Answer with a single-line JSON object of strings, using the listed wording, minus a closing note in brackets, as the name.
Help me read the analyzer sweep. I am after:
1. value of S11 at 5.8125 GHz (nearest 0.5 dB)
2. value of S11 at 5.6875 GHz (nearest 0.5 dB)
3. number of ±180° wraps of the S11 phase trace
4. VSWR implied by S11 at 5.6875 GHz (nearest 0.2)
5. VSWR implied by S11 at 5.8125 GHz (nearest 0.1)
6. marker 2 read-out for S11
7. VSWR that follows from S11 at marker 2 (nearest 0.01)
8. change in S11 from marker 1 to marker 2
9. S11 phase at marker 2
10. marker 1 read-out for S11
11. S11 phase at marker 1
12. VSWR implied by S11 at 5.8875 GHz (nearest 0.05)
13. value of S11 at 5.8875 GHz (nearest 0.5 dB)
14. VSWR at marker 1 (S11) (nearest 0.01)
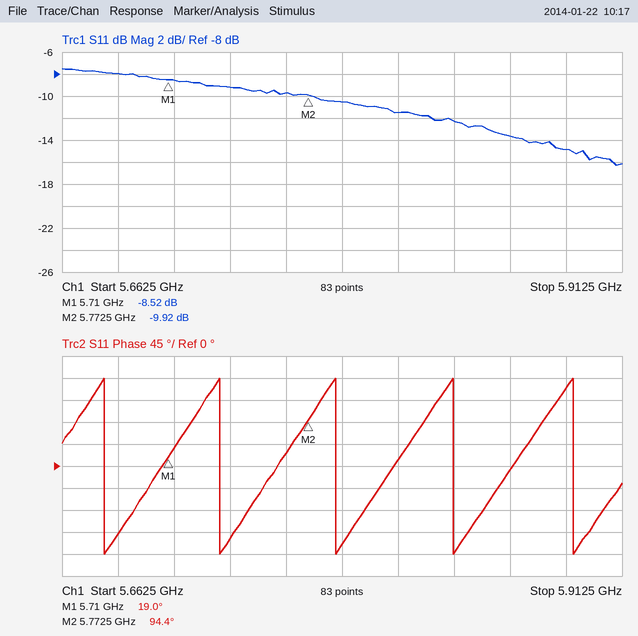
{"value of S11 at 5.8125 GHz": "-11.5 dB", "value of S11 at 5.6875 GHz": "-8.0 dB", "number of ±180° wraps of the S11 phase trace": "5", "VSWR implied by S11 at 5.6875 GHz": "2.4", "VSWR implied by S11 at 5.8125 GHz": "1.7", "marker 2 read-out for S11": "-9.92 dB", "VSWR that follows from S11 at marker 2": "1.94", "change in S11 from marker 1 to marker 2": "-1.40 dB", "S11 phase at marker 2": "94.4°", "marker 1 read-out for S11": "-8.52 dB", "S11 phase at marker 1": "19.0°", "VSWR implied by S11 at 5.8875 GHz": "1.45", "value of S11 at 5.8875 GHz": "-15.0 dB", "VSWR at marker 1 (S11)": "2.20"}
